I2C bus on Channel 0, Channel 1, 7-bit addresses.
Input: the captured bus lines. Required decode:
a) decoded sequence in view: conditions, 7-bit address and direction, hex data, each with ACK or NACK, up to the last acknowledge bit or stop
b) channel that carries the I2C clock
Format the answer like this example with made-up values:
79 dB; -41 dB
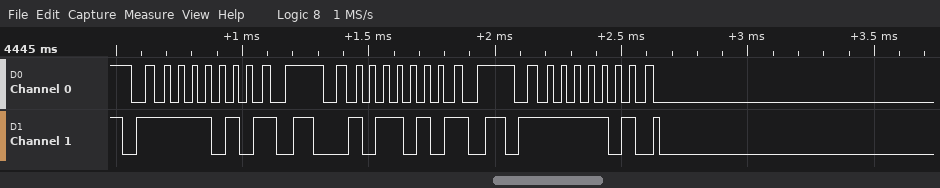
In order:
start, address 7D write NACK, stop, start, address 2D write NACK, stop, start, address 7E read ACK; Channel 0
